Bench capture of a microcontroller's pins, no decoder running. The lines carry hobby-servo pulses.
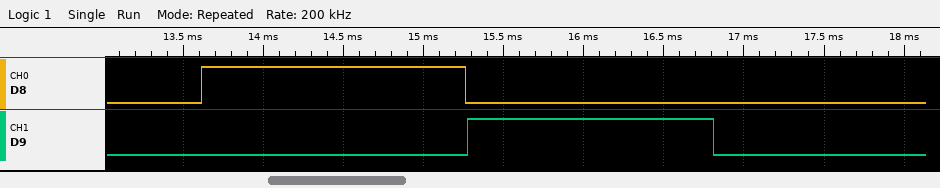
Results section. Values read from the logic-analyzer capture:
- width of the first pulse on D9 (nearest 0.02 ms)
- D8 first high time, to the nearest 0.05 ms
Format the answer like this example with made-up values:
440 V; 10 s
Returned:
1.54 ms; 1.65 ms
